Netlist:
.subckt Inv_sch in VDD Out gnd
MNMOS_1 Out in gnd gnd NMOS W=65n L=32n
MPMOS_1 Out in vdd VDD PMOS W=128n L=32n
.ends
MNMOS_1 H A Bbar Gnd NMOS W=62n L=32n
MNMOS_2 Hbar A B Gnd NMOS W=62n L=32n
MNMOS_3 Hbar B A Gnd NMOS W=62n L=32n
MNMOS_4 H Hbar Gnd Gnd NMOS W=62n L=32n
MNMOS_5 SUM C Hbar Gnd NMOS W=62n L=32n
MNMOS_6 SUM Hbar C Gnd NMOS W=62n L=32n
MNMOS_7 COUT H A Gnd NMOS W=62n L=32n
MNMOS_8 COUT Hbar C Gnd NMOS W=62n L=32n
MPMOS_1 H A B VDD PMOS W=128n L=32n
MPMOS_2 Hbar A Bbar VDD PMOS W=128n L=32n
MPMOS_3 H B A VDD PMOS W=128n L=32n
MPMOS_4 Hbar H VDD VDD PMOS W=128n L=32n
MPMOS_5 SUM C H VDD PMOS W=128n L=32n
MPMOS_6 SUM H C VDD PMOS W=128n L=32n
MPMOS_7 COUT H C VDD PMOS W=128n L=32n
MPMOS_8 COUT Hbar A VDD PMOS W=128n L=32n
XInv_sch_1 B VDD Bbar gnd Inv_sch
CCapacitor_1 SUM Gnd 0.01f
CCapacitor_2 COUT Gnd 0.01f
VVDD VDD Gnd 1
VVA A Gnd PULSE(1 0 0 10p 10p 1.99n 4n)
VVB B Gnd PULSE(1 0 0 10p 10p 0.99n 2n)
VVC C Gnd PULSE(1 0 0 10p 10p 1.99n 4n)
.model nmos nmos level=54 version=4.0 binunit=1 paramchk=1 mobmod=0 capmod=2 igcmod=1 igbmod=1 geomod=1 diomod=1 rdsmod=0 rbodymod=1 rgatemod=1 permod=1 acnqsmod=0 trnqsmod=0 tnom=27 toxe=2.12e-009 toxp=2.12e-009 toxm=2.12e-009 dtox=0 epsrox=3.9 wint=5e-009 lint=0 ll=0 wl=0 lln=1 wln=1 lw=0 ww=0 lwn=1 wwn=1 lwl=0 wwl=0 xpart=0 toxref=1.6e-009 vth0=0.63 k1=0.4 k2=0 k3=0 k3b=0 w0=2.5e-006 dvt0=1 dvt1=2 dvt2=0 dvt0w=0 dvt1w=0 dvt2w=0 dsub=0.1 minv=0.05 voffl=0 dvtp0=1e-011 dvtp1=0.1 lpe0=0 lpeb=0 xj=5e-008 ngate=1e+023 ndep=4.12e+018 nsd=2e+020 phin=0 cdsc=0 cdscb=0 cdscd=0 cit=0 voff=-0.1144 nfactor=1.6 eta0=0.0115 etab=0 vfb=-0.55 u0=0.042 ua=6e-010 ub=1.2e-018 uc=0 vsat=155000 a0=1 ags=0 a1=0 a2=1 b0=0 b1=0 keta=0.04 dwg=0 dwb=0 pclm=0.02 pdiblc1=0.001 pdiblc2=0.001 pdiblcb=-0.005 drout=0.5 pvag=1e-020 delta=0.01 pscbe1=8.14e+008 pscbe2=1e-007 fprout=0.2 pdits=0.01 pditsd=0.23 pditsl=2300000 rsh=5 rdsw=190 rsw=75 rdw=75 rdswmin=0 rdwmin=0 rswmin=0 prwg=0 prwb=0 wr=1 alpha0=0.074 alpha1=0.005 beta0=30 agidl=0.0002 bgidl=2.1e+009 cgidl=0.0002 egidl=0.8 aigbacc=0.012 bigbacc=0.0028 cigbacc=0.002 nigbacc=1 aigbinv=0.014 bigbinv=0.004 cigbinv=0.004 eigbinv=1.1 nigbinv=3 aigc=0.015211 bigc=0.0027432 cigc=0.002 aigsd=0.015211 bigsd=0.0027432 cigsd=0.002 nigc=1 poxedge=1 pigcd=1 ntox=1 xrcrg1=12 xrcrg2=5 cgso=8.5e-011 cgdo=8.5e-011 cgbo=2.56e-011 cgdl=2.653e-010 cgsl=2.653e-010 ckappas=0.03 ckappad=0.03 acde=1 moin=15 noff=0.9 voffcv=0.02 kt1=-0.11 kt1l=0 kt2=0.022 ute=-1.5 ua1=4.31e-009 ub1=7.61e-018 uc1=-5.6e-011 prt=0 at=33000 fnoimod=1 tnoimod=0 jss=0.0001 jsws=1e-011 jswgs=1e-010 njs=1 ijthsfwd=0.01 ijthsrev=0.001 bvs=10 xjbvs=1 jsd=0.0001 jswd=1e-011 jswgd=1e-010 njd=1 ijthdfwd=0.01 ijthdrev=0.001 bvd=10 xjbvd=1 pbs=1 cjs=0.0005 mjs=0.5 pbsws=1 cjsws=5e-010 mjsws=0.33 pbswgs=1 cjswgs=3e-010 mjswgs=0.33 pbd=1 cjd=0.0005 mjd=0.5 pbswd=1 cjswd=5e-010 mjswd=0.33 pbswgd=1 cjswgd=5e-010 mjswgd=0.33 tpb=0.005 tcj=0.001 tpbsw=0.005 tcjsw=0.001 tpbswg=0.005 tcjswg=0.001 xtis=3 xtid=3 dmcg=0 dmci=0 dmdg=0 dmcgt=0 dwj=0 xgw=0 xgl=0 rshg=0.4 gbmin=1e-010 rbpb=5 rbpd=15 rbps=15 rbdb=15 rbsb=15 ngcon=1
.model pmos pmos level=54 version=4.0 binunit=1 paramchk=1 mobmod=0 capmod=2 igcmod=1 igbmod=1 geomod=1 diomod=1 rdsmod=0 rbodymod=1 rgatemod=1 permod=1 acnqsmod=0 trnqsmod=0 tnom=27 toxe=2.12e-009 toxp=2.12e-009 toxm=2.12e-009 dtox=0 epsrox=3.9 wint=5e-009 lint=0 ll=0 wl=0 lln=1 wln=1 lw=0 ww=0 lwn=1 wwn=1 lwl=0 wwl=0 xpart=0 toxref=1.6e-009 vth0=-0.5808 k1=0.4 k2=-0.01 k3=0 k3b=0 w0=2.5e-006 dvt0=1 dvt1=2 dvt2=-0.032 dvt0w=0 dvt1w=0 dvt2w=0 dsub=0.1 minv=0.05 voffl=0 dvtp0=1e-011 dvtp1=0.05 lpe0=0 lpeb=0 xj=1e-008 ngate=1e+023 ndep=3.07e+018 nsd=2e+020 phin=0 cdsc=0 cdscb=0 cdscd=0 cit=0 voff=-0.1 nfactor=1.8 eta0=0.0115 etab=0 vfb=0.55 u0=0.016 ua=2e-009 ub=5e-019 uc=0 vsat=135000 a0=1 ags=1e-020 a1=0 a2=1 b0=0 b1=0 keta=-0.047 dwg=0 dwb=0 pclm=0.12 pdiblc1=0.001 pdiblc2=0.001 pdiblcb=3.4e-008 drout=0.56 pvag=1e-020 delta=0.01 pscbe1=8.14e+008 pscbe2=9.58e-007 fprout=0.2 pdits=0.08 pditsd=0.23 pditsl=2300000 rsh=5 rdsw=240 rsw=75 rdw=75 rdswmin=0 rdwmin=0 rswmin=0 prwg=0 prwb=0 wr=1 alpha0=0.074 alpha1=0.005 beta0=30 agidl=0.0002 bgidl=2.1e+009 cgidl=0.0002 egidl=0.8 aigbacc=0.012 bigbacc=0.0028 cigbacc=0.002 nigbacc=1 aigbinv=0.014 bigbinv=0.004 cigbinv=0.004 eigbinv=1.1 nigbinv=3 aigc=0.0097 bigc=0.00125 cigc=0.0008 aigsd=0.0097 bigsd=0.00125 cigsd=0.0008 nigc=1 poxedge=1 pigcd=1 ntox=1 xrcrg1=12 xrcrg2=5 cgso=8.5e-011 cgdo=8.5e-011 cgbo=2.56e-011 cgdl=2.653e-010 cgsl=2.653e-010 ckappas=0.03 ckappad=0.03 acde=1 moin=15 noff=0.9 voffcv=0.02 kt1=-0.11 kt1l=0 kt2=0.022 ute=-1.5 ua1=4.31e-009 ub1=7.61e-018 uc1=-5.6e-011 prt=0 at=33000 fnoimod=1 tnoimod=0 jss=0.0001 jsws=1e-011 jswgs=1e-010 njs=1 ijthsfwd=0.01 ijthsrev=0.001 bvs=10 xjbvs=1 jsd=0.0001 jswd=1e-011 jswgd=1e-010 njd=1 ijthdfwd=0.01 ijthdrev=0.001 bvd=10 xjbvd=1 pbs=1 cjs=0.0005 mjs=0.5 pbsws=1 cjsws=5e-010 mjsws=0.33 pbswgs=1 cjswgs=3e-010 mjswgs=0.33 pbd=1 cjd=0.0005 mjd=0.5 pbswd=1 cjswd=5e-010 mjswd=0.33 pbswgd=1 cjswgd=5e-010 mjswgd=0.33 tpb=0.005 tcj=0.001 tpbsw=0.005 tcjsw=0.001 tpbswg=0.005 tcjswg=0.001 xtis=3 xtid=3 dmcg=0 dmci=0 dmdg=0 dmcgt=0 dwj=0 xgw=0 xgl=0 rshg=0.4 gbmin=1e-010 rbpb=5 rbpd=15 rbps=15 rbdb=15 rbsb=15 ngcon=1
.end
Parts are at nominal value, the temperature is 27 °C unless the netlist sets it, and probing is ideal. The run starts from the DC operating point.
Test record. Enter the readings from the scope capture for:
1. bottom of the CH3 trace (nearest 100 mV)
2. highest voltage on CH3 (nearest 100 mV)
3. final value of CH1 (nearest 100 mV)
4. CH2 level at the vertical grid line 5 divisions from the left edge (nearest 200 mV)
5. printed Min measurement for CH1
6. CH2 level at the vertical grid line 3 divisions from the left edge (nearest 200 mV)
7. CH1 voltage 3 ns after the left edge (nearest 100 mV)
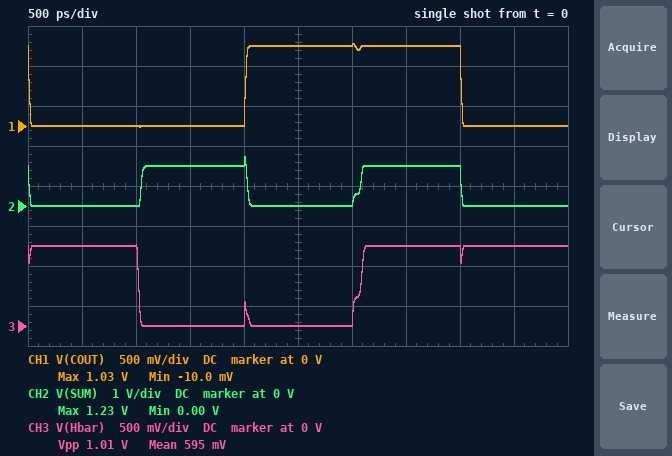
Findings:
0 V
1.0 V
0 V
0 V
-10.0 mV
1.0 V
1.0 V
